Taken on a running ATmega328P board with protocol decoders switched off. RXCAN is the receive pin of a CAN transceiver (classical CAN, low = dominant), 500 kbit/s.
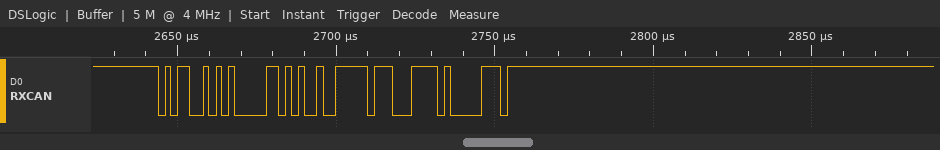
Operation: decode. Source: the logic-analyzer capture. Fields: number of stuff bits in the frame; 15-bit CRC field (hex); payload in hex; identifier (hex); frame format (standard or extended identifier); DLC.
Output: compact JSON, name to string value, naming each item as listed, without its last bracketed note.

{"number of stuff bits in the frame": "3", "15-bit CRC field": "0x0F41", "payload in hex": "A4 FF", "identifier": "0x595", "frame format": "standard", "DLC": "2"}
